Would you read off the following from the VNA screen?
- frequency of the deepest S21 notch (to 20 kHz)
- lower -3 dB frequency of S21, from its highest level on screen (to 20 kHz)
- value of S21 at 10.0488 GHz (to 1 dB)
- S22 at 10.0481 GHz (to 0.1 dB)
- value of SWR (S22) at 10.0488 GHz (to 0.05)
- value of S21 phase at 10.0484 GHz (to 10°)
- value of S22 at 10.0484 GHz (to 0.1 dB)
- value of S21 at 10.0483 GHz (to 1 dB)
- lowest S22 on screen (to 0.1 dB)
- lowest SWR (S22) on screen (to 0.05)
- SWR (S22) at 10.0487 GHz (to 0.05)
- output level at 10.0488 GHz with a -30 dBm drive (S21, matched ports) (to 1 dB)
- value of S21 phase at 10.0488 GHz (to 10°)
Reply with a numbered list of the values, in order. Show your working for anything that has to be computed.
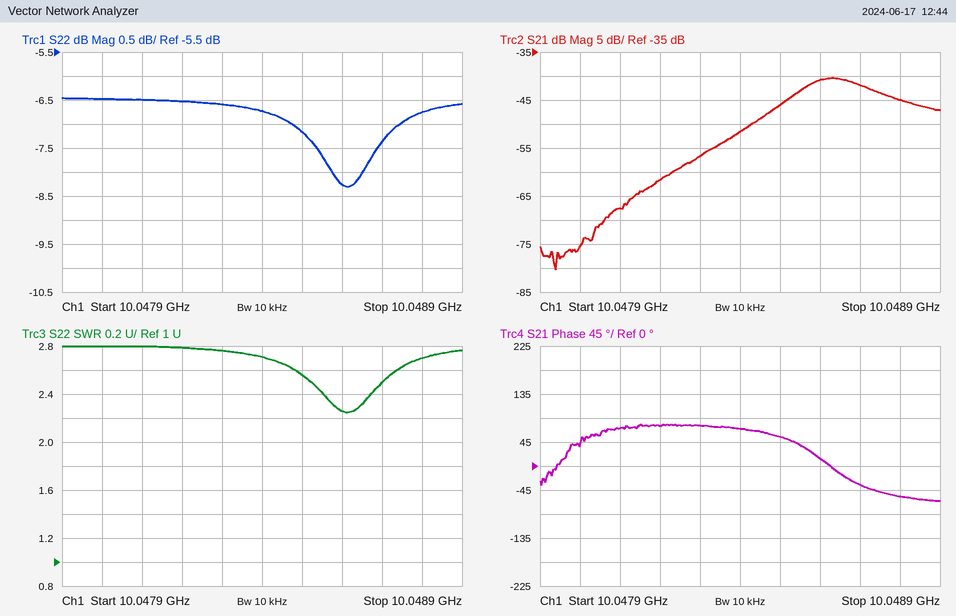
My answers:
1. 10.04794 GHz
2. 10.04854 GHz
3. -45 dB
4. -6.5 dB
5. 2.70
6. 70°
7. -6.7 dB
8. -57 dB
9. -8.3 dB
10. 2.25
11. 2.50
12. -30 dBm + (-45 dB) = -75 dBm
13. -60°
